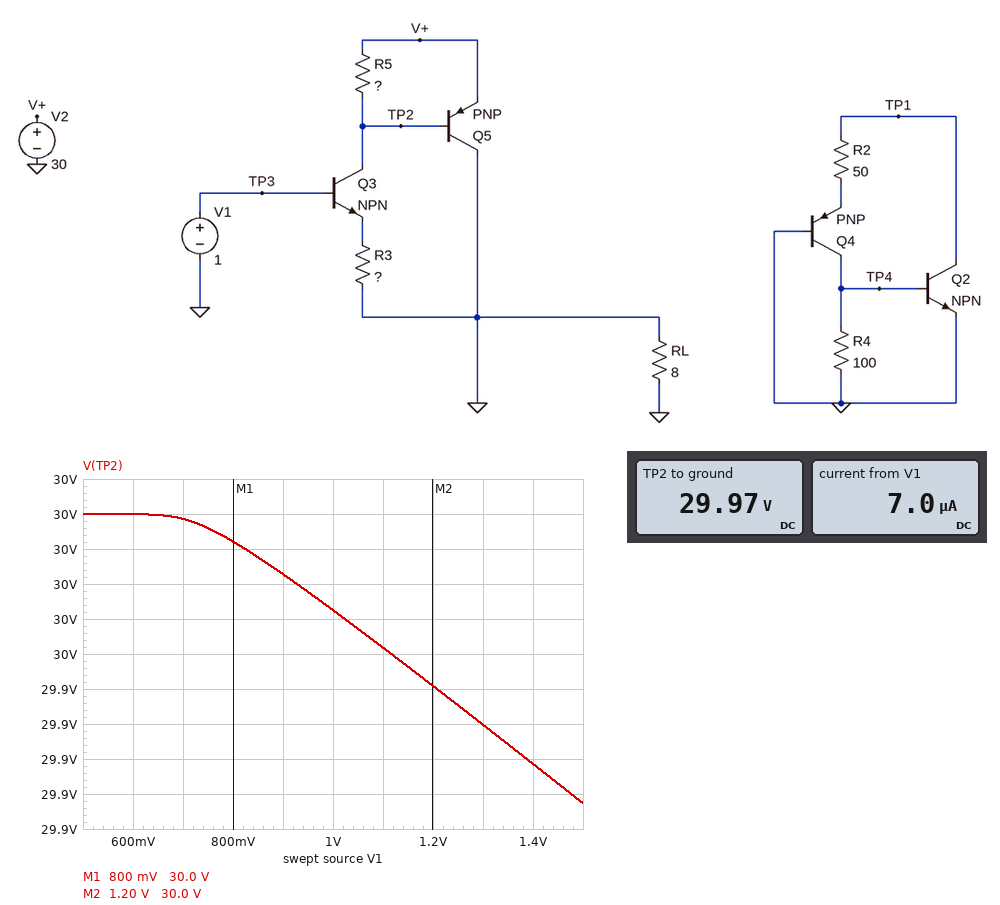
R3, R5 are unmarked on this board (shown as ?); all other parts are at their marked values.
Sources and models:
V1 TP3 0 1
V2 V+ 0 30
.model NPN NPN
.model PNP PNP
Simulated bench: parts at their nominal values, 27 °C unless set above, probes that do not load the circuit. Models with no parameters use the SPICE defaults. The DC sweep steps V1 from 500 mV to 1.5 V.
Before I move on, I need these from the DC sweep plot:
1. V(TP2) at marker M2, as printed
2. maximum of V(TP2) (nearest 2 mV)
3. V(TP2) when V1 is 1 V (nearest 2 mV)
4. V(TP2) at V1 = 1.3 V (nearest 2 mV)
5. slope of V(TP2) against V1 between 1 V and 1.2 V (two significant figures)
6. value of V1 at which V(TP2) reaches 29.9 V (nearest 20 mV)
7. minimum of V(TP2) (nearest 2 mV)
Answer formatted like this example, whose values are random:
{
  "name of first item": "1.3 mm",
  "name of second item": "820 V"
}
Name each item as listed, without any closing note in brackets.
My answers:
{
  "V(TP2) at marker M2, as printed": "30.0 V",
  "maximum of V(TP2)": "30.000 V",
  "V(TP2) when V1 is 1 V": "29.972 V",
  "V(TP2) at V1 = 1.3 V": "29.940 V",
  "slope of V(TP2) against V1 between 1 V and 1.2 V": "-0.11 V/V",
  "value of V1 at which V(TP2) reaches 29.9 V": "1.30 V",
  "minimum of V(TP2)": "29.918 V"
}
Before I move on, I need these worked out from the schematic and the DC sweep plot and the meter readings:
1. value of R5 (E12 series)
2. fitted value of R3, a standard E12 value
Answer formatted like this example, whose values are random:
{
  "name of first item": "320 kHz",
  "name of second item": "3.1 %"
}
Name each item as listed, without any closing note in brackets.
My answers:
{
  "value of R5": "39 Ω",
  "fitted value of R3, a standard E12 value": "330 Ω"
}
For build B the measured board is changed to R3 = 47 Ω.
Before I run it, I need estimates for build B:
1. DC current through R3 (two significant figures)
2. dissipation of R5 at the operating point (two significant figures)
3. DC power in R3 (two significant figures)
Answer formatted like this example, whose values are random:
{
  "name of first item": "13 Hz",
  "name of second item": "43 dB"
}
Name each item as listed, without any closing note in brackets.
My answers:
{
  "DC current through R3": "4.0 mA",
  "dissipation of R5 at the operating point": "620 µW",
  "DC power in R3": "770 µW"
}
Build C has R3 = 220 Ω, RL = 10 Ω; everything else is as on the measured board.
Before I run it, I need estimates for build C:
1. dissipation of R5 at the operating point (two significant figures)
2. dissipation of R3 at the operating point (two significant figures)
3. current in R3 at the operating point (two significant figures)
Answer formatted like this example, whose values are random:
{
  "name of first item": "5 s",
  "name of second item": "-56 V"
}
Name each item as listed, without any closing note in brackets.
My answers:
{
  "dissipation of R5 at the operating point": "40 µW",
  "dissipation of R3 at the operating point": "230 µW",
  "current in R3 at the operating point": "1.0 mA"
}
